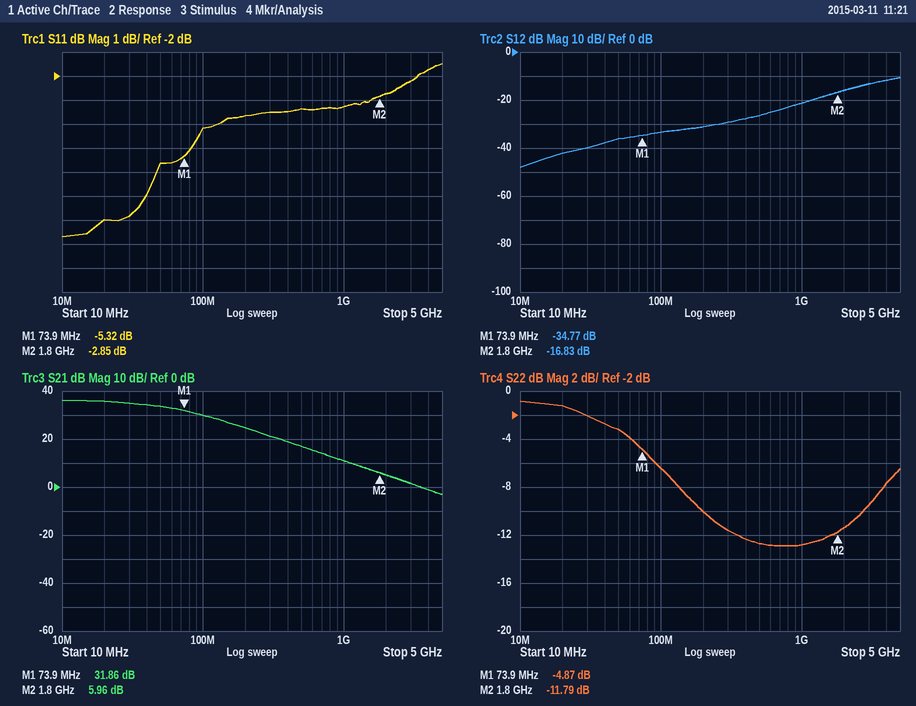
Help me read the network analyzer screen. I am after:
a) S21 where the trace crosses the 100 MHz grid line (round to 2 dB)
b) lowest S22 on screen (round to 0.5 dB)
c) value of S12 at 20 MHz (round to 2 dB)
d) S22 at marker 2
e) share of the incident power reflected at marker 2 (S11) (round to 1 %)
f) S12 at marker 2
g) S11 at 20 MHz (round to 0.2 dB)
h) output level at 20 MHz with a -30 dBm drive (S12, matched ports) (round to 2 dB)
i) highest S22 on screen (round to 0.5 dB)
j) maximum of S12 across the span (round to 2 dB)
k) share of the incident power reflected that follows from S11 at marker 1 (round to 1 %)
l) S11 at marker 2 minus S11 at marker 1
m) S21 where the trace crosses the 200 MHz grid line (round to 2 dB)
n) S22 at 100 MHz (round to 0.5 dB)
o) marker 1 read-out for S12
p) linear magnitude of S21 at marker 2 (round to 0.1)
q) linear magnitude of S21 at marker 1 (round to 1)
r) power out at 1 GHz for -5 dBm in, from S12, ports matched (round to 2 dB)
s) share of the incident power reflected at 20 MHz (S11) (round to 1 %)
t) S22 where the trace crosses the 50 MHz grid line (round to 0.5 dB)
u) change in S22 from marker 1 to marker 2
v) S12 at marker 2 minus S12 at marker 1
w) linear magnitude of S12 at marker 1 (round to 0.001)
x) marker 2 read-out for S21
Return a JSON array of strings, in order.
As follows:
["30 dB", "-13.0 dB", "-42 dB", "-11.79 dB", "52 %", "-16.83 dB", "-8.0 dB", "-72 dBm", "-1.0 dB", "-10 dB", "29 %", "2.47 dB", "24 dB", "-6.5 dB", "-34.77 dB", "2.0", "39", "-26 dBm", "16 %", "-3.0 dB", "-6.92 dB", "17.94 dB", "0.018", "5.96 dB"]
